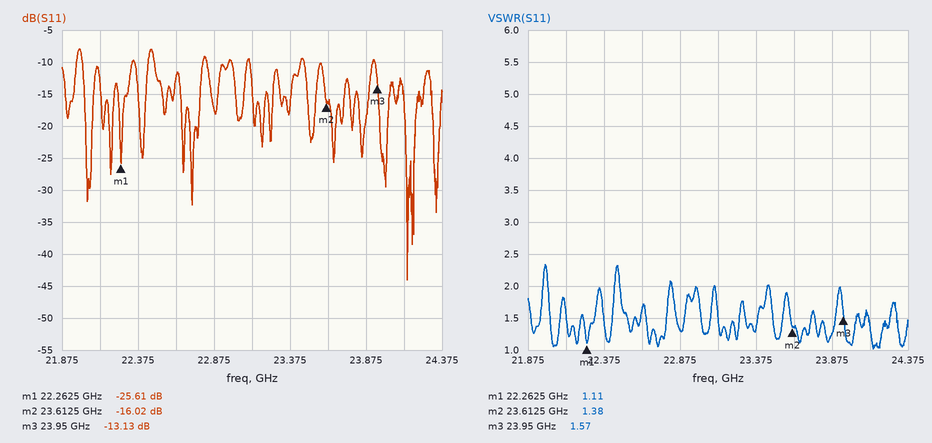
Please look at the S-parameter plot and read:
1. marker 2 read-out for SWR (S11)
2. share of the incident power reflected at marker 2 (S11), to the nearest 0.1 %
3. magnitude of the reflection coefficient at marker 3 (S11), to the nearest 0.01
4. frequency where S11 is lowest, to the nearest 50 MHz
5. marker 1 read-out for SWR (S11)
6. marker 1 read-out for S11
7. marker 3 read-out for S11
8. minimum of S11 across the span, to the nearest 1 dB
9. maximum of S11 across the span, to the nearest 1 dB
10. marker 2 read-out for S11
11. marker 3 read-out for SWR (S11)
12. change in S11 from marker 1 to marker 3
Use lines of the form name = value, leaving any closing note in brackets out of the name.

marker 2 read-out for SWR = 1.38
share of the incident power reflected at marker 2 (S11), to the nearest 0.1 % = 2.5 %
magnitude of the reflection coefficient at marker 3 (S11), to the nearest 0.01 = 0.22
frequency where S11 is lowest, to the nearest 50 MHz = 24.15 GHz
marker 1 read-out for SWR = 1.11
marker 1 read-out for S11 = -25.61 dB
marker 3 read-out for S11 = -13.13 dB
minimum of S11 across the span, to the nearest 1 dB = -44 dB
maximum of S11 across the span, to the nearest 1 dB = -8 dB
marker 2 read-out for S11 = -16.02 dB
marker 3 read-out for SWR = 1.57
change in S11 from marker 1 to marker 3 = 12.48 dB
